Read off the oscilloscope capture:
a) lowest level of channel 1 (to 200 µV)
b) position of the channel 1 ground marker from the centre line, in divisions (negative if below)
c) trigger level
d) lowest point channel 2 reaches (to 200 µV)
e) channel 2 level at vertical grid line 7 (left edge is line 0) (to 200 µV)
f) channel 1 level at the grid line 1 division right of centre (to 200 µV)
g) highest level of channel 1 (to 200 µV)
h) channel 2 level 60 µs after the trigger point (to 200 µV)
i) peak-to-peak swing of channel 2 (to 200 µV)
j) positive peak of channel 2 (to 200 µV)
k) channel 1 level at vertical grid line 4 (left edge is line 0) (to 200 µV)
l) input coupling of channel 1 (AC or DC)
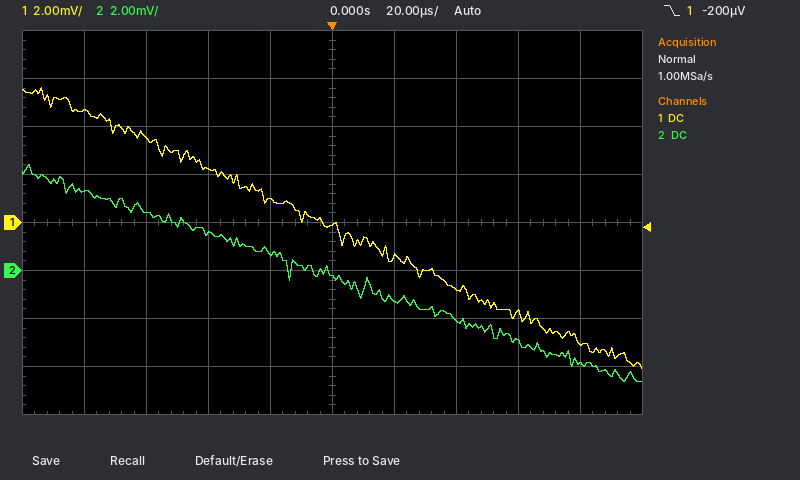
-6.0 mV
0.0 div
-200 µV
-4.6 mV
-2.0 mV
-1.4 mV
5.6 mV
-3.0 mV
9.0 mV
4.4 mV
1.0 mV
DC
